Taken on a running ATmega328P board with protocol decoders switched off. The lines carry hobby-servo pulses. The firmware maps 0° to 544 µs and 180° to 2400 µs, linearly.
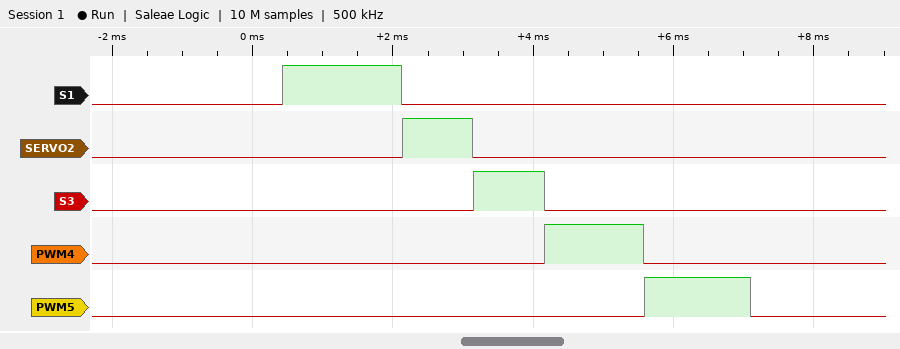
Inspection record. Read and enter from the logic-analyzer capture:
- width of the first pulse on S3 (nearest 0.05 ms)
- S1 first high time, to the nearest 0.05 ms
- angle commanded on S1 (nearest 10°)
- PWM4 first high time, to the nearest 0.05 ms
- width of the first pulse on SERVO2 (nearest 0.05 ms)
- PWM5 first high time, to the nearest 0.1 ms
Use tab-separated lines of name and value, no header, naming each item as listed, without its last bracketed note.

width of the first pulse on S3	1.00 ms
S1 first high time, to the nearest 0.05 ms	1.70 ms
angle commanded on S1	110°
PWM4 first high time, to the nearest 0.05 ms	1.40 ms
width of the first pulse on SERVO2	1.00 ms
PWM5 first high time, to the nearest 0.1 ms	1.5 ms
